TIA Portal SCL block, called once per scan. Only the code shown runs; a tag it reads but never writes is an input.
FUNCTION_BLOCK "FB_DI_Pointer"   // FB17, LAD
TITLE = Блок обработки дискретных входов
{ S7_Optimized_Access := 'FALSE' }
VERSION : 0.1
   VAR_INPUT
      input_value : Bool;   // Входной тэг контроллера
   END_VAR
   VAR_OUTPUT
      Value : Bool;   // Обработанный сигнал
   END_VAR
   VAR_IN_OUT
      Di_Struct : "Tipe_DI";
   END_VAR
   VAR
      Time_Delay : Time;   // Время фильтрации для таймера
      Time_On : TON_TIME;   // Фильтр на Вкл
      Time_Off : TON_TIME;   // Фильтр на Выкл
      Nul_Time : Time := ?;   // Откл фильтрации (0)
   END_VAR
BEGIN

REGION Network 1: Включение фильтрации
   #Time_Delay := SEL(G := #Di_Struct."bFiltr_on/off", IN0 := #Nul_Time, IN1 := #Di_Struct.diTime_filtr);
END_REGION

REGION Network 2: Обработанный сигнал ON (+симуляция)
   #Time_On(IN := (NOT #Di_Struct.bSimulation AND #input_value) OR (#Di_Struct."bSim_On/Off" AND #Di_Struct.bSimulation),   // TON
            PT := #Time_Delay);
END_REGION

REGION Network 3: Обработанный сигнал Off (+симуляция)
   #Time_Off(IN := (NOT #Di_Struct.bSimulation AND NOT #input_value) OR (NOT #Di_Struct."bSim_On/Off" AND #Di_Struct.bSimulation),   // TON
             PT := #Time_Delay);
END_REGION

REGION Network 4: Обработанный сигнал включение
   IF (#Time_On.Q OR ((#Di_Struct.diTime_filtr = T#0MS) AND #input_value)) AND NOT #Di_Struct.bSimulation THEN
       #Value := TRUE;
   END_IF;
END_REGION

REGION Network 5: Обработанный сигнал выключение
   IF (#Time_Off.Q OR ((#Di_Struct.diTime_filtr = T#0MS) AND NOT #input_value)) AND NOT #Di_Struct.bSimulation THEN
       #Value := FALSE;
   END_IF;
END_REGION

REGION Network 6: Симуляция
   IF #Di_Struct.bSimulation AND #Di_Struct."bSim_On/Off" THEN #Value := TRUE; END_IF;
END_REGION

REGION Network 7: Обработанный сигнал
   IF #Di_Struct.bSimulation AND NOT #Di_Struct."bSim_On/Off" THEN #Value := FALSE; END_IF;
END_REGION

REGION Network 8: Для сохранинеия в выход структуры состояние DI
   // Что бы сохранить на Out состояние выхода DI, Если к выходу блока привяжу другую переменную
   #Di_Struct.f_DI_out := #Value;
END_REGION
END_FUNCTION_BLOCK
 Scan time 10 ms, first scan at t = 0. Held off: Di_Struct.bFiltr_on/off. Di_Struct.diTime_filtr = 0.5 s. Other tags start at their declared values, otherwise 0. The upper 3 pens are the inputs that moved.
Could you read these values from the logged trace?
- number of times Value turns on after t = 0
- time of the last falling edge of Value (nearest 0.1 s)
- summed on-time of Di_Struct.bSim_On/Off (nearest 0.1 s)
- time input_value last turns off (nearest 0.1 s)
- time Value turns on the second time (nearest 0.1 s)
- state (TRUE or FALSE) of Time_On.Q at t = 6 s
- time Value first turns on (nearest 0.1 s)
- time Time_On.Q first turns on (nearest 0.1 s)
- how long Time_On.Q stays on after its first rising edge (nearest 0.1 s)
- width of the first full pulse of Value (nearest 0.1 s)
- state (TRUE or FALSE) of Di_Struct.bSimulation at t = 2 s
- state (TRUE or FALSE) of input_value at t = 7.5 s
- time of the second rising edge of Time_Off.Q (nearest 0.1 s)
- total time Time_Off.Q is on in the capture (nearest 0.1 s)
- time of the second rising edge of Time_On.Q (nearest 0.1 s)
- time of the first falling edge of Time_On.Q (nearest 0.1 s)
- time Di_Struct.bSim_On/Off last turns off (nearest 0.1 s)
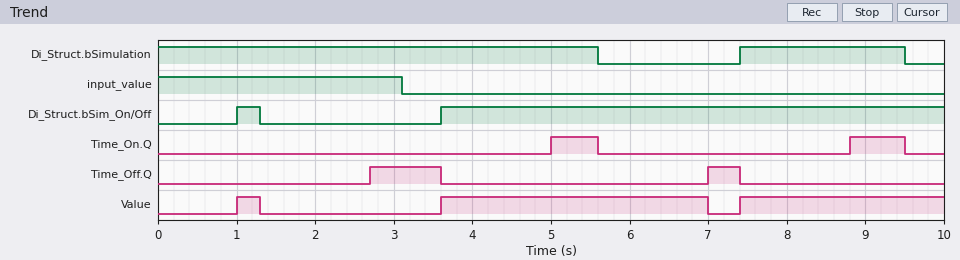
3
7.0 s
6.7 s
3.1 s
3.6 s
FALSE
1.0 s
5.0 s
0.6 s
0.3 s
TRUE
FALSE
7.0 s
1.3 s
8.8 s
5.6 s
1.3 s
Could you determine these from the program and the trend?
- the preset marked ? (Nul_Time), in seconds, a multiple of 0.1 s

1.4 s
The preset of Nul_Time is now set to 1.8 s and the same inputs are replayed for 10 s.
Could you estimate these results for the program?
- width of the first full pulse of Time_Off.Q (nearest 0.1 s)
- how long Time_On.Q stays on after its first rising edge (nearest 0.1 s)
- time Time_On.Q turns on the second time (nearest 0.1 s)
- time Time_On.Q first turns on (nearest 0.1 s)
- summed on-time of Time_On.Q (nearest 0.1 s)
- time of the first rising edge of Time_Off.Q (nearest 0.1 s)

0.5 s
0.2 s
9.2 s
5.4 s
0.5 s
3.1 s
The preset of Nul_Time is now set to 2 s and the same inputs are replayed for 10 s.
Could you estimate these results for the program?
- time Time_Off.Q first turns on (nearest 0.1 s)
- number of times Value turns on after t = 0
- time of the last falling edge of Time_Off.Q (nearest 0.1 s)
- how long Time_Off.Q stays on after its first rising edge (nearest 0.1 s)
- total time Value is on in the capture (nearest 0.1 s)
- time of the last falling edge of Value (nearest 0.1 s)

3.3 s
2
3.6 s
0.3 s
6.7 s
1.3 s
